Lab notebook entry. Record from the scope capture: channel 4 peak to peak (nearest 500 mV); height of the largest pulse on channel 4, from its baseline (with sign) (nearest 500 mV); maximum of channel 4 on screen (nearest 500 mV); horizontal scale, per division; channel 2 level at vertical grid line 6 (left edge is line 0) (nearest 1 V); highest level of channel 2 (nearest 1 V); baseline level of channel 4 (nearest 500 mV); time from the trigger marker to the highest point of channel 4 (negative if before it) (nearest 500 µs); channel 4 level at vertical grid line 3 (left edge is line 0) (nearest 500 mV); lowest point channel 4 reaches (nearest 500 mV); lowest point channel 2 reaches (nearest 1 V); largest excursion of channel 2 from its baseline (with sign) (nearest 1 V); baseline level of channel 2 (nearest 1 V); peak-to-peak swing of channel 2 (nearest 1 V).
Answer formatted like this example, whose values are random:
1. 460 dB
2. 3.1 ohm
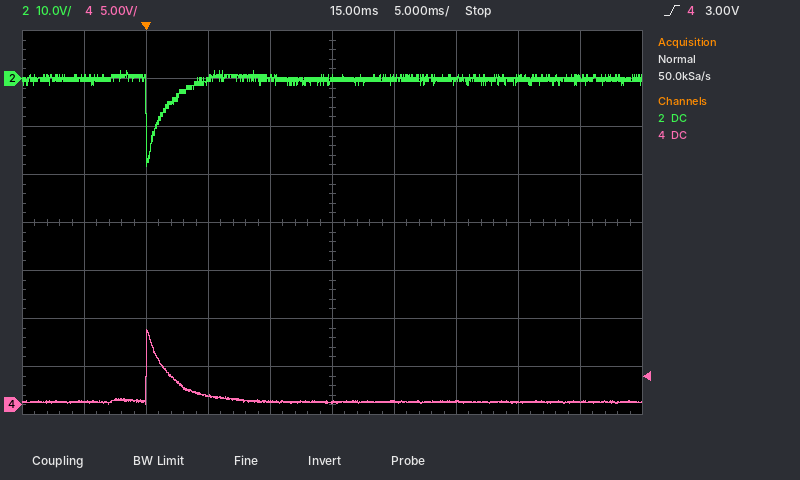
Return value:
1. 8.0 V
2. +7.5 V
3. 8.0 V
4. 5 ms
5. 0 V
6. 2 V
7. 500 mV
8. 0.0 ms
9. 1.0 V
10. 0.0 V
11. -18 V
12. -18 V
13. 0 V
14. 20 V
